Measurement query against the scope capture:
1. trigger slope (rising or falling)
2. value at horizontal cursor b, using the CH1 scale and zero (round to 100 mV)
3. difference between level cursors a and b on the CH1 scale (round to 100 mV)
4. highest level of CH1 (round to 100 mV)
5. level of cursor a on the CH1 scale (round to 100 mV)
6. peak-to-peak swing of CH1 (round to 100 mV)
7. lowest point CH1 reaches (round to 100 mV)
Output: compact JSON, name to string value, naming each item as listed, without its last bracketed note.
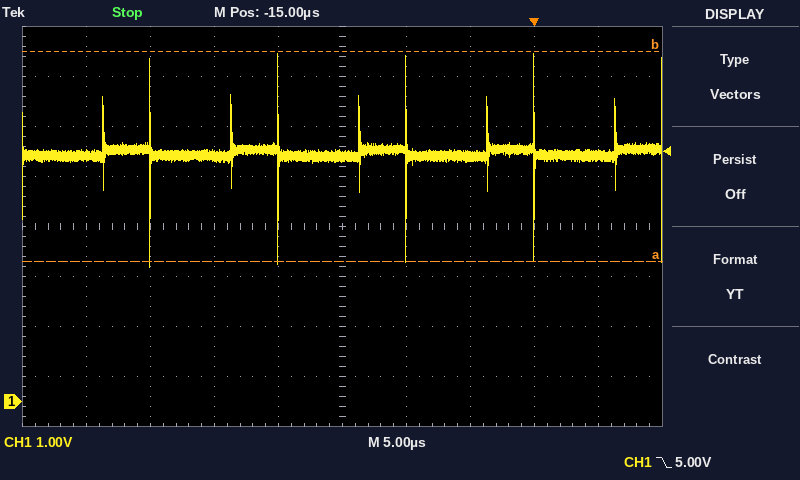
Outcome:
{"trigger slope": "falling", "value at horizontal cursor b, using the CH1 scale and zero": "7.0 V", "difference between level cursors a and b on the CH1 scale": "4.2 V", "highest level of CH1": "7.0 V", "level of cursor a on the CH1 scale": "2.8 V", "peak-to-peak swing of CH1": "4.3 V", "lowest point CH1 reaches": "2.7 V"}
